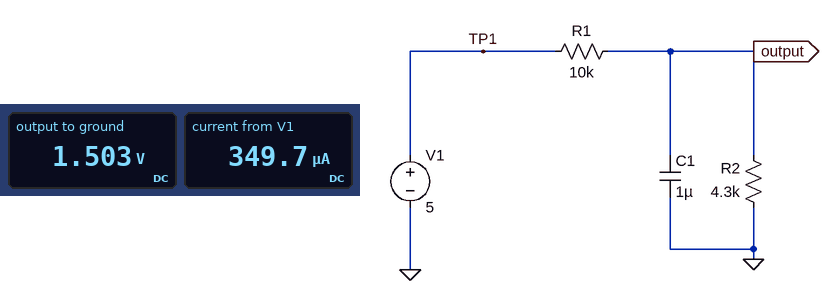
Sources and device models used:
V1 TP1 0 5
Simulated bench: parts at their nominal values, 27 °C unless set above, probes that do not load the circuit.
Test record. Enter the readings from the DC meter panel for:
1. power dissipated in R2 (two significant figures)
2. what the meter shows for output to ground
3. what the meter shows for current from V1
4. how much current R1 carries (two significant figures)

530 µW
1.503 V
349.7 µA
350 µA
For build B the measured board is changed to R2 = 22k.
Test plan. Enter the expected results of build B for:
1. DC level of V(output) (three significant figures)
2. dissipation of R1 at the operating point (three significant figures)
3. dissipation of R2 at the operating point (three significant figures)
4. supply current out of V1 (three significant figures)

3.44 V
244 µW
537 µW
156 µA
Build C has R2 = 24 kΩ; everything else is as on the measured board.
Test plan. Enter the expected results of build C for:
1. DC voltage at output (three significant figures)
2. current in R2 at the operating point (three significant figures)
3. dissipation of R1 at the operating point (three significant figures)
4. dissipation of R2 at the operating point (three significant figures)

3.53 V
147 µA
216 µW
519 µW
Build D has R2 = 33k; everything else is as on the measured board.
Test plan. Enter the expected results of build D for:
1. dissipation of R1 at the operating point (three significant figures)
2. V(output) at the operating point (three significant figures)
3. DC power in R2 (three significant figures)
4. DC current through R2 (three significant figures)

135 µW
3.84 V
446 µW
116 µA
